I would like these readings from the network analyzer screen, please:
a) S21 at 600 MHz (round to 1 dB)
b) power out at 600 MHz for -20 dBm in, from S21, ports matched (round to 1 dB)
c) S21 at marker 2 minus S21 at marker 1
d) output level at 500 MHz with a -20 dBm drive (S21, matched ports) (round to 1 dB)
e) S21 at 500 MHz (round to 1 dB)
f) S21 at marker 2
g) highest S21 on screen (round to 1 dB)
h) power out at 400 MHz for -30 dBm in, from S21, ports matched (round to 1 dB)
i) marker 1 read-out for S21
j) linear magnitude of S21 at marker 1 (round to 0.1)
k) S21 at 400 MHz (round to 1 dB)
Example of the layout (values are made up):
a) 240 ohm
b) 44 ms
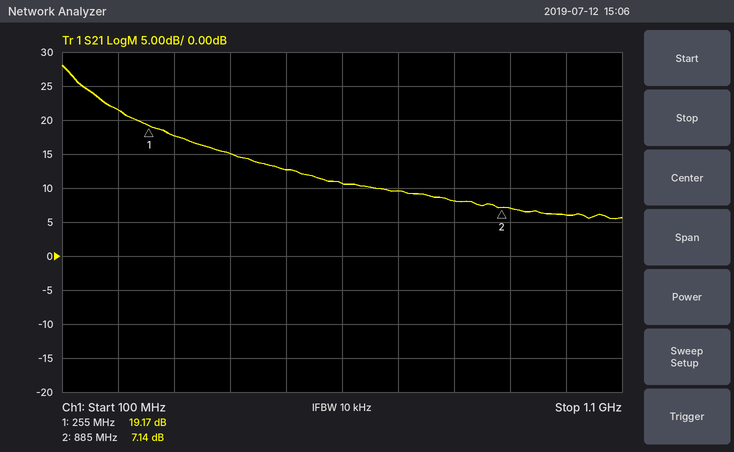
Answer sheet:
a) 11 dB
b) -9 dBm
c) -12.03 dB
d) -7 dBm
e) 13 dB
f) 7.14 dB
g) 28 dB
h) -15 dBm
i) 19.17 dB
j) 9.1
k) 15 dB
